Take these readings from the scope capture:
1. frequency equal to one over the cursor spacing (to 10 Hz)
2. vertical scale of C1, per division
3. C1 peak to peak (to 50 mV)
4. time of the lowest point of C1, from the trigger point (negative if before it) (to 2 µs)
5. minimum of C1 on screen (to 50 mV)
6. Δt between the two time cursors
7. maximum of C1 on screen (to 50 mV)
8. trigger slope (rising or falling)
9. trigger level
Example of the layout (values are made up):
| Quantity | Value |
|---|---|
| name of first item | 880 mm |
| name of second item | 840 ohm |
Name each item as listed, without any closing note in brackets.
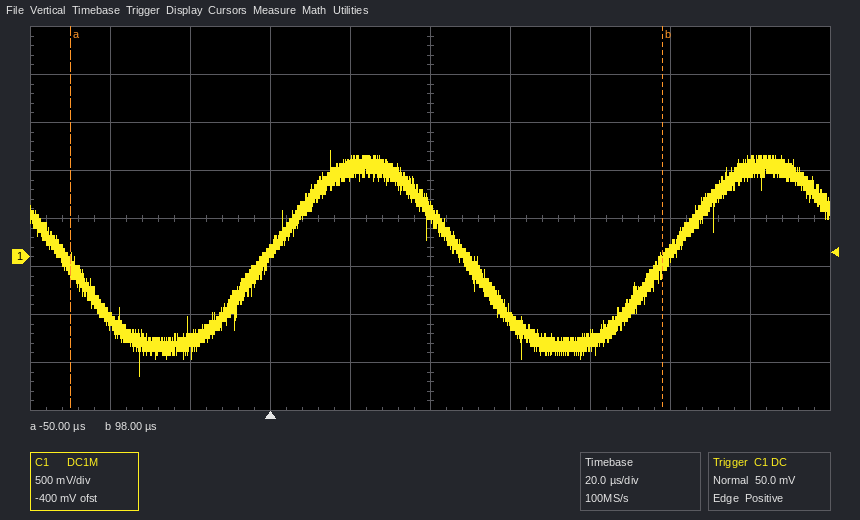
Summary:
| Quantity | Value |
|---|---|
| frequency equal to one over the cursor spacing | 6.76 kHz |
| vertical scale of C1, per division | 500 mV |
| C1 peak to peak | 2.35 V |
| time of the lowest point of C1, from the trigger point (negative if before it) | -32 µs |
| minimum of C1 on screen | -1.25 V |
| Δt between the two time cursors | 148 µs |
| maximum of C1 on screen | 1.10 V |
| trigger slope | rising |
| trigger level | 50.0 mV |
